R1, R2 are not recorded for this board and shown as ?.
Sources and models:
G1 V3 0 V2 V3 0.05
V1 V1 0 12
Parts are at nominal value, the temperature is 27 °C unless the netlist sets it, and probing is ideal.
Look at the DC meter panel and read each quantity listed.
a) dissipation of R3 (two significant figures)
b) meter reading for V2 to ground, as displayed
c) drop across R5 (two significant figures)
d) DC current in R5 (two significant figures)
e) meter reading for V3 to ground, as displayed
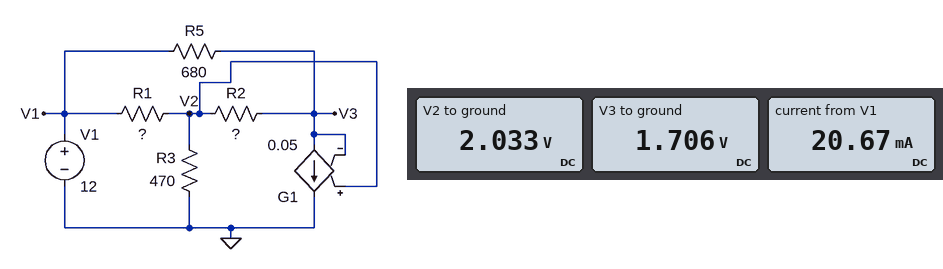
8.8 mW
2.033 V
10 V
15 mA
1.706 V
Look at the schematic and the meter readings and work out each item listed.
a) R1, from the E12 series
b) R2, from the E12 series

1.8 kΩ
270 Ω
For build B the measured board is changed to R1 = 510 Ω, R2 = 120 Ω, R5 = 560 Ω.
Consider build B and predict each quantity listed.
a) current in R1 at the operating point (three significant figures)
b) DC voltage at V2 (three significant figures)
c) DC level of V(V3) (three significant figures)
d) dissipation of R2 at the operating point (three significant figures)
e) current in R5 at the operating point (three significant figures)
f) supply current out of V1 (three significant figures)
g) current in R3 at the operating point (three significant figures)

13.5 mA
5.13 V
4.82 V
789 µW
12.8 mA
26.3 mA
10.9 mA
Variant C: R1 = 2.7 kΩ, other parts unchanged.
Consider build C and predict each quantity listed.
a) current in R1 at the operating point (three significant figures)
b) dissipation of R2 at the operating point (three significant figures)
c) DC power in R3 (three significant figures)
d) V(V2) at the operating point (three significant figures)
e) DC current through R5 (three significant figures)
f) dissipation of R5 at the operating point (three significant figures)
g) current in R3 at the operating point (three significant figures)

3.98 mA
460 µW
3.36 mW
1.26 V
16.3 mA
181 mW
2.67 mA
